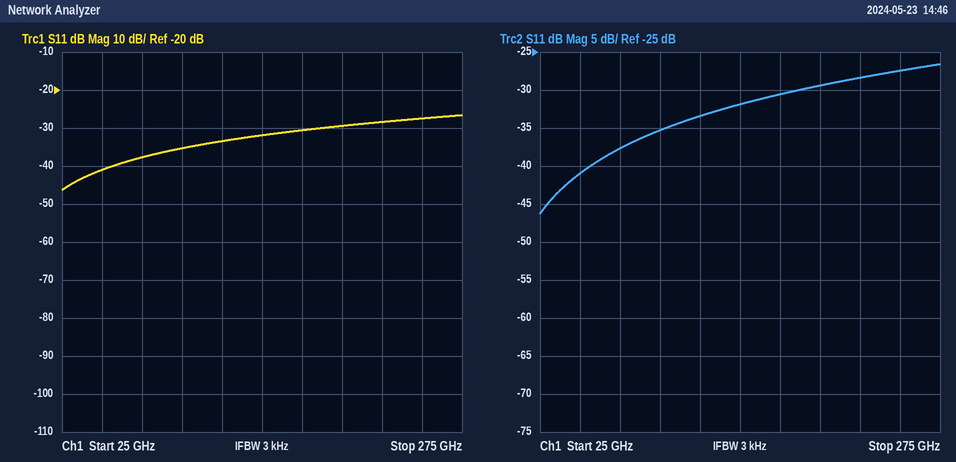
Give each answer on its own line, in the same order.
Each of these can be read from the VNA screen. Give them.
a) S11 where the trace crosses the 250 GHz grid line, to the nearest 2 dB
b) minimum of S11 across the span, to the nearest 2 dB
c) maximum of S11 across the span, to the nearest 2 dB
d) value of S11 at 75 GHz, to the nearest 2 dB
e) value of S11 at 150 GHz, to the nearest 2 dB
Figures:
-28 dB
-46 dB
-26 dB
-38 dB
-32 dB
